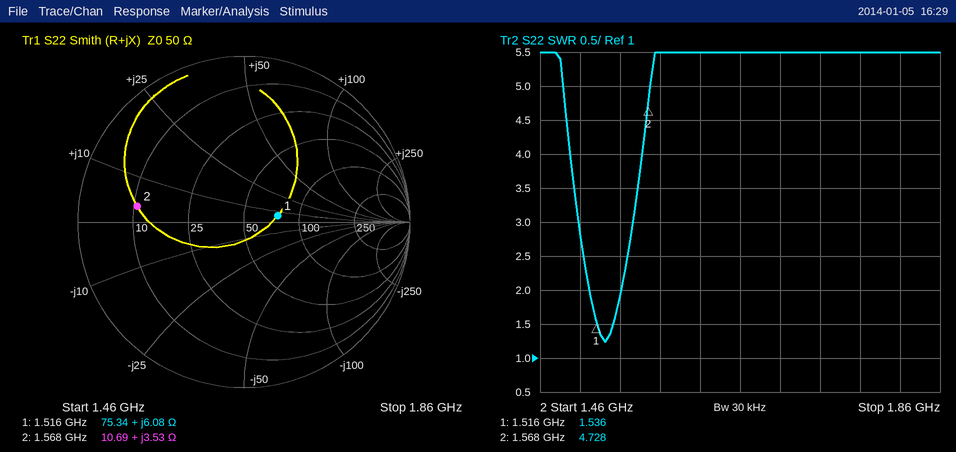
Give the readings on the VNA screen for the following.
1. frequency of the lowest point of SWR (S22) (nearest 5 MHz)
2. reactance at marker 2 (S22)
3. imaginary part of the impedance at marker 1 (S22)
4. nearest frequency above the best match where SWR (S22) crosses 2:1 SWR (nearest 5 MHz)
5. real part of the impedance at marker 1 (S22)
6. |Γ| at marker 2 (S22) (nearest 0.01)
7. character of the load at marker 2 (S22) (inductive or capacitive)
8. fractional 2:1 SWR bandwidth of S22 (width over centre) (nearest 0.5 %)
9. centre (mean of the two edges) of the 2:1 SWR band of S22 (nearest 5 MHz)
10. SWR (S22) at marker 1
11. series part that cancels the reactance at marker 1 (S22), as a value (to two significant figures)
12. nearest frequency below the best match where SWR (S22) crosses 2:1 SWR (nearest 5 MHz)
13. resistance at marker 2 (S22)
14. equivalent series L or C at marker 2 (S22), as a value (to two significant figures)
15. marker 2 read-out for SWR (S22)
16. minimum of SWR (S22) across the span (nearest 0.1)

1.525 GHz
+3.53 Ω
+6.08 Ω
1.540 GHz
75.34 Ω
0.65
inductive
2.0 %
1.525 GHz
1.536
17 pF
1.510 GHz
10.69 Ω
360 pH
4.728
1.2
